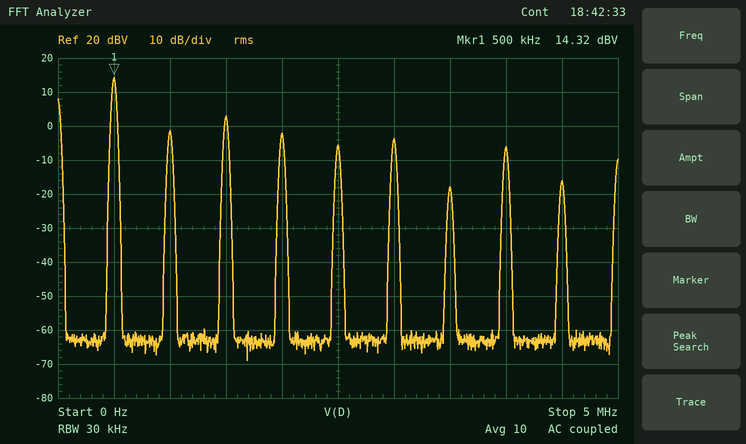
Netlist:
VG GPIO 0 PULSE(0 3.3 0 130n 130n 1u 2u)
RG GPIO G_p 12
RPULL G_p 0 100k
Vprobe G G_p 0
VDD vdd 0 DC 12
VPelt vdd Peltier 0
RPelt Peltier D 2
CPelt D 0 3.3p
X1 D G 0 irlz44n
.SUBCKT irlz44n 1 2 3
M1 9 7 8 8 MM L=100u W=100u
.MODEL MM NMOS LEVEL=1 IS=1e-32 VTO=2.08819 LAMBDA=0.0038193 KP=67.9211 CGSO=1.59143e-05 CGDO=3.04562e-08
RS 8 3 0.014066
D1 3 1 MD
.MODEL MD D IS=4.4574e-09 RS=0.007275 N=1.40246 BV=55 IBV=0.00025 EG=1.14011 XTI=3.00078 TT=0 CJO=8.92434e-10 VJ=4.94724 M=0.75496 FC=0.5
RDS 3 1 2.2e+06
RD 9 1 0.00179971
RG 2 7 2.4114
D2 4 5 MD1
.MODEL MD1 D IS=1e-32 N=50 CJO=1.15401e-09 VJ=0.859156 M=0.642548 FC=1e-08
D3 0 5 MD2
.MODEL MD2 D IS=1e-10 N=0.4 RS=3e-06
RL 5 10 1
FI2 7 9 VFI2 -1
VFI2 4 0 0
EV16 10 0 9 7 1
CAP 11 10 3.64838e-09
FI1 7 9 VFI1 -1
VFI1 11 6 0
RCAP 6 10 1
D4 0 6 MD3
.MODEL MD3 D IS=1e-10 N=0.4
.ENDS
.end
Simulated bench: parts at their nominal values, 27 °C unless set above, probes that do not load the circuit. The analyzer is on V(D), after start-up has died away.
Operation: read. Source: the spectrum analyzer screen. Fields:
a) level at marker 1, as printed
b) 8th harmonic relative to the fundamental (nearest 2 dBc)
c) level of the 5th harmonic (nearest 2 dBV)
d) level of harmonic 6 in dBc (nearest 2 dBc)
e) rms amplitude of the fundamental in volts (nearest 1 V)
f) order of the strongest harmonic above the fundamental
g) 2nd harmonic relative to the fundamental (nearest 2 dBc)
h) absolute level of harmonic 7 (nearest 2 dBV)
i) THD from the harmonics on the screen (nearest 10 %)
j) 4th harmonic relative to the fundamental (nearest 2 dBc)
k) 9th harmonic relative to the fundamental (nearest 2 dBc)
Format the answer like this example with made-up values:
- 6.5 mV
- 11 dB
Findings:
- 14.32 dBV
- -20 dBc
- -6 dBV
- -18 dBc
- 5 V
- 3
- -16 dBc
- -18 dBV
- 40 %
- -16 dBc
- -30 dBc
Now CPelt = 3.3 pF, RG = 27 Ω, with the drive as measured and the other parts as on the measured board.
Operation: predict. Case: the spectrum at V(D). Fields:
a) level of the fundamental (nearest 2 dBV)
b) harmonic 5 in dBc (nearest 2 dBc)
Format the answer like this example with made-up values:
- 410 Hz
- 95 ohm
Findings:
- 14 dBV
- -26 dBc
